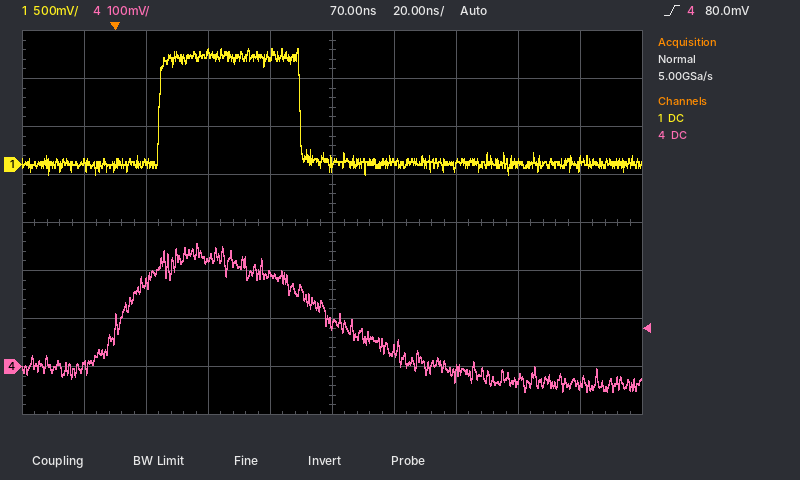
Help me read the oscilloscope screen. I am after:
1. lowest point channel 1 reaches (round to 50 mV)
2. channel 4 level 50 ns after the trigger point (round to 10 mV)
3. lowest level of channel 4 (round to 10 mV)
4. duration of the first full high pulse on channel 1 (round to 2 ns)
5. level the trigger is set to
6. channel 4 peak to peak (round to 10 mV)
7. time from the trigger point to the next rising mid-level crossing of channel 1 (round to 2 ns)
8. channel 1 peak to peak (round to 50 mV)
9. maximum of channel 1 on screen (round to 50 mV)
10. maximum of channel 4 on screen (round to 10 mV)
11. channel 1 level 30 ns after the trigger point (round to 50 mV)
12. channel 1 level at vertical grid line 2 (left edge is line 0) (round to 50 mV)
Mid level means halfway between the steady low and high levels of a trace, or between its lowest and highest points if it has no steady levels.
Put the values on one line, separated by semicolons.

-100 mV; 190 mV; -50 mV; 46 ns; 80.0 mV; 310 mV; 14 ns; 1.30 V; 1.20 V; 260 mV; 1.15 V; 0 mV
